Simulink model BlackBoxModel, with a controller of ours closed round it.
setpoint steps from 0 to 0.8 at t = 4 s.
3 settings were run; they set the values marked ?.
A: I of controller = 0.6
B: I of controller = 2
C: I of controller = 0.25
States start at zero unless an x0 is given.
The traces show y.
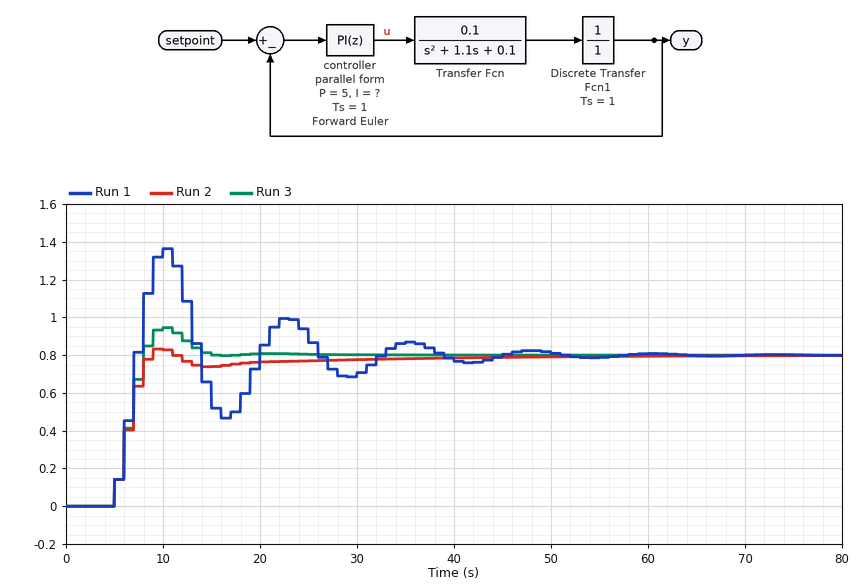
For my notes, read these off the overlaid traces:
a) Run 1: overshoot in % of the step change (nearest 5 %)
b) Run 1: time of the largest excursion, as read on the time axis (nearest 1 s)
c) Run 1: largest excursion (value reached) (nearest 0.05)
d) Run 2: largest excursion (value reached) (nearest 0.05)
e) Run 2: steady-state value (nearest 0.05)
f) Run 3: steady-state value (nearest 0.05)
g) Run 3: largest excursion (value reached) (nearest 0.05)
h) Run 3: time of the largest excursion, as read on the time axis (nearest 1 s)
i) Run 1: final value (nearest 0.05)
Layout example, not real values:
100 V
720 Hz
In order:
70 %
10 s
1.35
0.85
0.80
0.80
0.95
10 s
0.80
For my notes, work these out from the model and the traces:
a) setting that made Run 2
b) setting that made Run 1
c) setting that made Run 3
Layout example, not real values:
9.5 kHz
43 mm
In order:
C
B
A
